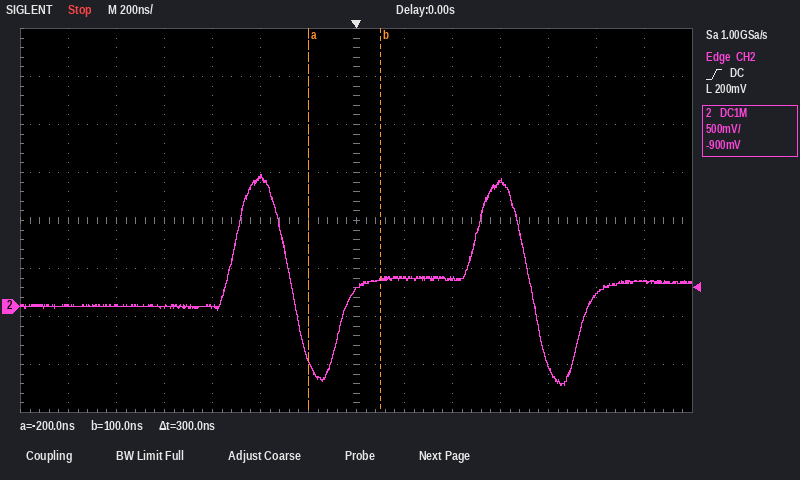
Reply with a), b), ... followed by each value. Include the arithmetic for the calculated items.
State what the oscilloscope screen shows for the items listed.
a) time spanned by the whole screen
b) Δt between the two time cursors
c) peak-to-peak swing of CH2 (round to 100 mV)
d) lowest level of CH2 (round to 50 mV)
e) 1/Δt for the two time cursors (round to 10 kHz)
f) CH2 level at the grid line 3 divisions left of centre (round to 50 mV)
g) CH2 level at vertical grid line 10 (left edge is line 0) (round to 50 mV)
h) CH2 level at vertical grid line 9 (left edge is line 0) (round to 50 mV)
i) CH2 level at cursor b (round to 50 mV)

a) 2.8 µs
b) 300 ns
c) 2.20 V
d) -800 mV
e) 1 / 300 ns ≈ 3.33 MHz
f) 0 mV
g) 1.30 V
h) 300 mV
i) 300 mV
